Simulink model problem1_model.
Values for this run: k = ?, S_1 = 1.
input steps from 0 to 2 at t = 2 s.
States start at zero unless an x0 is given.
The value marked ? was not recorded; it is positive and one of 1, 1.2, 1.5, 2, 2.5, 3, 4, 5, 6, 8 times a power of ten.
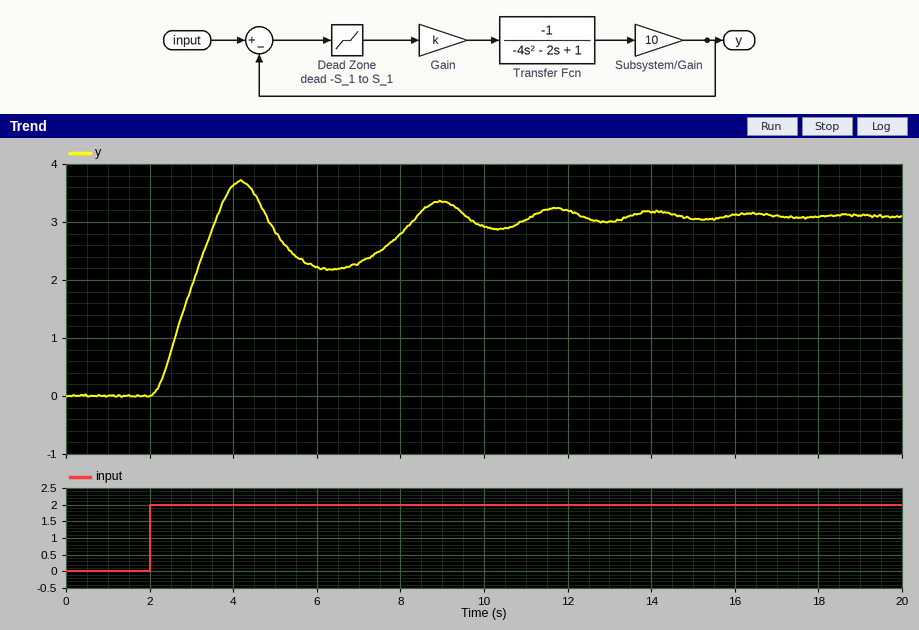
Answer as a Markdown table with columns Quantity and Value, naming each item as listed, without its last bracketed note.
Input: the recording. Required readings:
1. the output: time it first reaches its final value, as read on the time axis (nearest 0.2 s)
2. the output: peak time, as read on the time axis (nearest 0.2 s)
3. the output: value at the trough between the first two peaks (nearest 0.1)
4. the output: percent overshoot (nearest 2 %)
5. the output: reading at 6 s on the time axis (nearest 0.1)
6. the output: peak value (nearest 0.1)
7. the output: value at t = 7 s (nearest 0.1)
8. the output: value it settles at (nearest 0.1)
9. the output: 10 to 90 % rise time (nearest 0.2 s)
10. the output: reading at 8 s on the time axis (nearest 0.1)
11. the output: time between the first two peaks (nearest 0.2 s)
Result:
| Quantity | Value |
|---|---|
| the output: time it first reaches its final value, as read on the time axis | 3.6 s |
| the output: peak time, as read on the time axis | 4.2 s |
| the output: value at the trough between the first two peaks | 2.2 |
| the output: percent overshoot | 20 % |
| the output: reading at 6 s on the time axis | 2.2 |
| the output: peak value | 3.7 |
| the output: value at t = 7 s | 2.3 |
| the output: value it settles at | 3.1 |
| the output: 10 to 90 % rise time | 1.2 s |
| the output: reading at 8 s on the time axis | 2.8 |
| the output: time between the first two peaks | 4.8 s |
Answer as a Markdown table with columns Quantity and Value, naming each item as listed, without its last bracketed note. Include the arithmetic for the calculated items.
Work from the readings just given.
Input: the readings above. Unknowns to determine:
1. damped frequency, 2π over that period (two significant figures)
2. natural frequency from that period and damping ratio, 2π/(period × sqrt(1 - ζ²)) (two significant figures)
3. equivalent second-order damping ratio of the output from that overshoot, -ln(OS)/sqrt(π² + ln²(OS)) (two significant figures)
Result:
| Quantity | Value |
|---|---|
| damped frequency, 2π over that period | 2π / 4.8 = 1.3 rad/s |
| natural frequency from that period and damping ratio, 2π/(period × sqrt(1 - ζ²)) | 2π / (4.8 × sqrt(1 - 0.46²)) = 1.5 rad/s |
| equivalent second-order damping ratio of the output from that overshoot, -ln(OS)/sqrt(π² + ln²(OS)) | ln(0.2) = -1.609; 1.609 / sqrt(9.870 + 2.590) = 0.46 |
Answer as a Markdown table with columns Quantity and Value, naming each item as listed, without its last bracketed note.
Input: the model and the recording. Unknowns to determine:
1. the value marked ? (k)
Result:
| Quantity | Value |
|---|---|
| the value marked ? | 3 |
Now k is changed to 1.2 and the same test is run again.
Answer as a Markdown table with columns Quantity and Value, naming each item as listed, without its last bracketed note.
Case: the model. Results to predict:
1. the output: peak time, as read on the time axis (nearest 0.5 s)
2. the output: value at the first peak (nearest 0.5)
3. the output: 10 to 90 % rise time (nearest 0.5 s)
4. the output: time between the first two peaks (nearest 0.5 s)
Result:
| Quantity | Value |
|---|---|
| the output: peak time, as read on the time axis | 5.5 s |
| the output: value at the first peak | 4.0 |
| the output: 10 to 90 % rise time | 2.0 s |
| the output: time between the first two peaks | 4.0 s |
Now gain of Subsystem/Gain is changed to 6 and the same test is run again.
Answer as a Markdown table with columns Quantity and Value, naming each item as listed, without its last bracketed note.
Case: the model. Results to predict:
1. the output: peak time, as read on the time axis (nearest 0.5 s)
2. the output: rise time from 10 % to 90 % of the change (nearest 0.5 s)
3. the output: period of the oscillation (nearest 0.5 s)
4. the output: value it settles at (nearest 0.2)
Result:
| Quantity | Value |
|---|---|
| the output: peak time, as read on the time axis | 5.0 s |
| the output: rise time from 10 % to 90 % of the change | 1.5 s |
| the output: period of the oscillation | 4.0 s |
| the output: value it settles at | 3.2 |
